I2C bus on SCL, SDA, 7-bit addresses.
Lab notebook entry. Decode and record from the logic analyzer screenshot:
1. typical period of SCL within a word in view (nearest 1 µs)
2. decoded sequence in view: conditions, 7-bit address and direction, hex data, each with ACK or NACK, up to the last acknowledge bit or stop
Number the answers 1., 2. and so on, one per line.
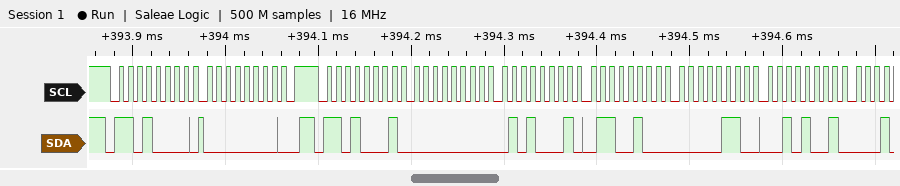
1. 10 µs
2. start, address 68 write ACK, 00 ACK, stop, start, address 68 read ACK, 00 ACK, 51 ACK, 64 ACK, 06 ACK, 29 ACK
